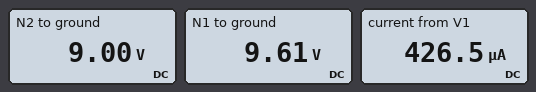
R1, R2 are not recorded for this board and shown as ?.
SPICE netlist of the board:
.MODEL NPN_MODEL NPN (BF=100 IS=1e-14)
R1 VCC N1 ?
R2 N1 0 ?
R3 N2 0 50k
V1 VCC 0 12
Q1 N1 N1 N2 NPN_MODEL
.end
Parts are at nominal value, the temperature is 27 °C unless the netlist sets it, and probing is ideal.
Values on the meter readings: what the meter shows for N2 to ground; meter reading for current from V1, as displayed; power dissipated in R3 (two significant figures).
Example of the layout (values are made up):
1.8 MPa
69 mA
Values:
9.00 V
426.5 µA
1.6 mW
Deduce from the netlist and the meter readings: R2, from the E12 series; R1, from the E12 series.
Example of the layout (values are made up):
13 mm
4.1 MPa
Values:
39 kΩ
5.6 kΩ
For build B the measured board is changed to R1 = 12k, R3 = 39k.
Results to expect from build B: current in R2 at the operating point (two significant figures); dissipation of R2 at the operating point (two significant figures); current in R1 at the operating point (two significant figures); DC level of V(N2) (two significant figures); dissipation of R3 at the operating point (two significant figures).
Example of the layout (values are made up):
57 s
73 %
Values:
190 µA
1.5 mW
370 µA
6.9 V
1.2 mW
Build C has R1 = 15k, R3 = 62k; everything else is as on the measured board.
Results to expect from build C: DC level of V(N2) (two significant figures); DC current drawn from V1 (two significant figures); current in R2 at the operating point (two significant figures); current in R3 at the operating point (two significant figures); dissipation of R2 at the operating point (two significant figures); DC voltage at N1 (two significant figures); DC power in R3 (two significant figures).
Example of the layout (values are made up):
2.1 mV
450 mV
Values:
6.9 V
300 µA
190 µA
110 µA
1.4 mW
7.5 V
760 µW
